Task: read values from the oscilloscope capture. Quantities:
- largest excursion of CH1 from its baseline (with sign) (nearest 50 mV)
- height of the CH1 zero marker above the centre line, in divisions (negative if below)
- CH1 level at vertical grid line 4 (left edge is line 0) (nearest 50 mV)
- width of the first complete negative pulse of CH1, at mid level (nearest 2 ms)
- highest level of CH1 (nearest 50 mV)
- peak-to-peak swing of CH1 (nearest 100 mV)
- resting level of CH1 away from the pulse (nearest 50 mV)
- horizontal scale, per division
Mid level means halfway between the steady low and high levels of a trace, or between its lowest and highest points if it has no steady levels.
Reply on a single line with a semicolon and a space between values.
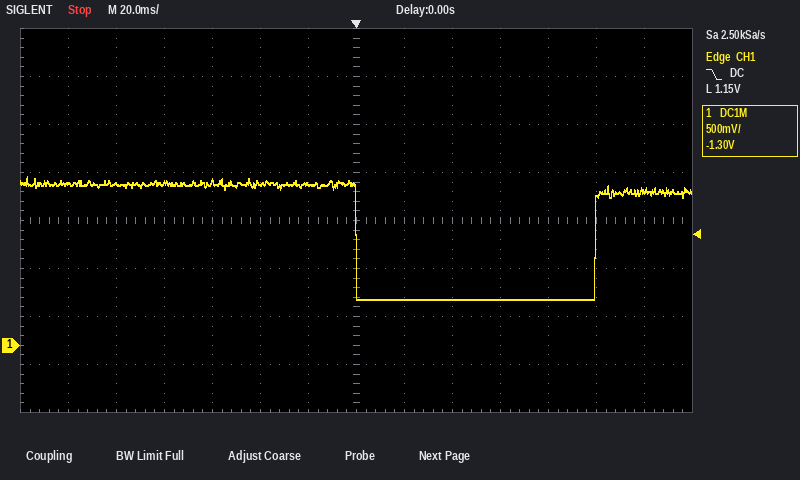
-1.20 V; -2.6 div; 1.70 V; 100 ms; 1.75 V; 1.30 V; 1.65 V; 20 ms
